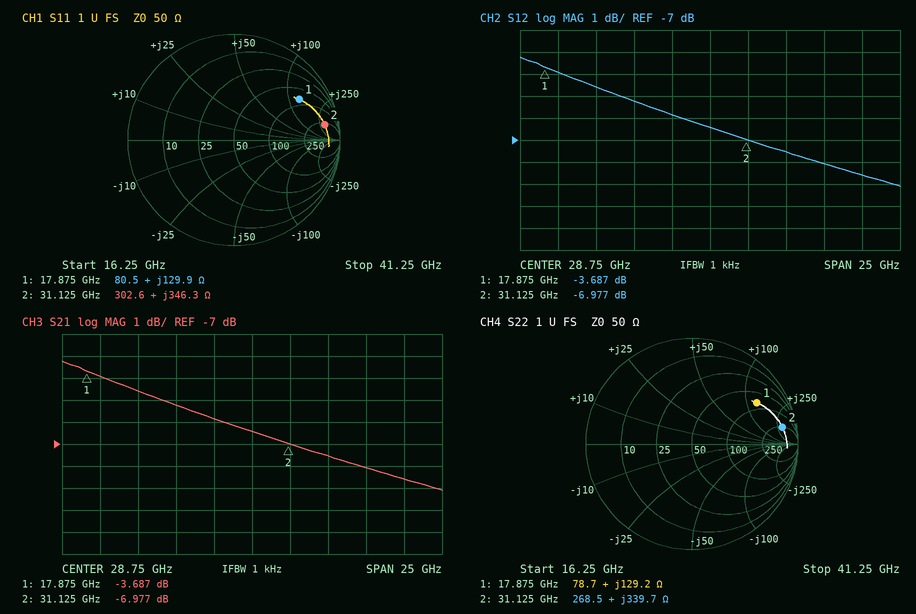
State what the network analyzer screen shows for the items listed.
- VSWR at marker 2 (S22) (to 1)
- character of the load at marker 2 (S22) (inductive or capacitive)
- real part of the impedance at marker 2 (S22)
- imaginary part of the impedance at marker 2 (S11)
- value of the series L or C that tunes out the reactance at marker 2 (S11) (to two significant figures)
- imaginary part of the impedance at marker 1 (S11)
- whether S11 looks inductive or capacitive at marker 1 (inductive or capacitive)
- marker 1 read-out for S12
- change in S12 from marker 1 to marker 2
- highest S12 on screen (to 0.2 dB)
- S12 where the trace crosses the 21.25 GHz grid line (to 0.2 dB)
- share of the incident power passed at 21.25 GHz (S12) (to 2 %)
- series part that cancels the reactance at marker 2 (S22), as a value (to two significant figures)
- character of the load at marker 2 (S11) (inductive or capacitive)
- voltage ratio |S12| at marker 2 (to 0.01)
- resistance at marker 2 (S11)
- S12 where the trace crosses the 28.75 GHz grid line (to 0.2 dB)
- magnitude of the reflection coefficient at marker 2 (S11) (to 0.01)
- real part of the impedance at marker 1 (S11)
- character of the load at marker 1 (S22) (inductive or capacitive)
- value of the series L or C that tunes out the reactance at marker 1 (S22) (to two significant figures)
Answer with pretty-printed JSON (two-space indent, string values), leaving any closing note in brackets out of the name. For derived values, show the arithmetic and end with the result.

{
  "VSWR at marker 2 (S22)": "14",
  "character of the load at marker 2 (S22)": "inductive",
  "real part of the impedance at marker 2": "268.5 Ω",
  "imaginary part of the impedance at marker 2": "+346.3 Ω",
  "value of the series L or C that tunes out the reactance at marker 2 (S11)": "C = 1/(2π × 31.125 GHz × 346.3 Ω) ≈ 15 fF",
  "imaginary part of the impedance at marker 1": "+129.9 Ω",
  "whether S11 looks inductive or capacitive at marker 1": "inductive",
  "marker 1 read-out for S12": "-3.687 dB",
  "change in S12 from marker 1 to marker 2": "-6.977 − (-3.687) = -3.290 dB",
  "highest S12 on screen": "-3.2 dB",
  "S12 where the trace crosses the 21.25 GHz grid line": "-4.6 dB",
  "share of the incident power passed at 21.25 GHz (S12)": "10^(-4.6/10) ≈ 34.7 %, so 34 % to the nearest 2 %",
  "series part that cancels the reactance at marker 2 (S22), as a value": "C = 1/(2π × 31.125 GHz × 339.7 Ω) ≈ 15 fF",
  "character of the load at marker 2 (S11)": "inductive",
  "voltage ratio |S12| at marker 2": "10^(-6.977/20) ≈ 0.45",
  "resistance at marker 2": "302.6 Ω",
  "S12 where the trace crosses the 28.75 GHz grid line": "-6.4 dB",
  "magnitude of the reflection coefficient at marker 2 (S11)": "0.87",
  "real part of the impedance at marker 1": "80.5 Ω",
  "character of the load at marker 1 (S22)": "inductive",
  "value of the series L or C that tunes out the reactance at marker 1 (S22)": "C = 1/(2π × 17.875 GHz × 129.2 Ω) ≈ 69 fF"
}
